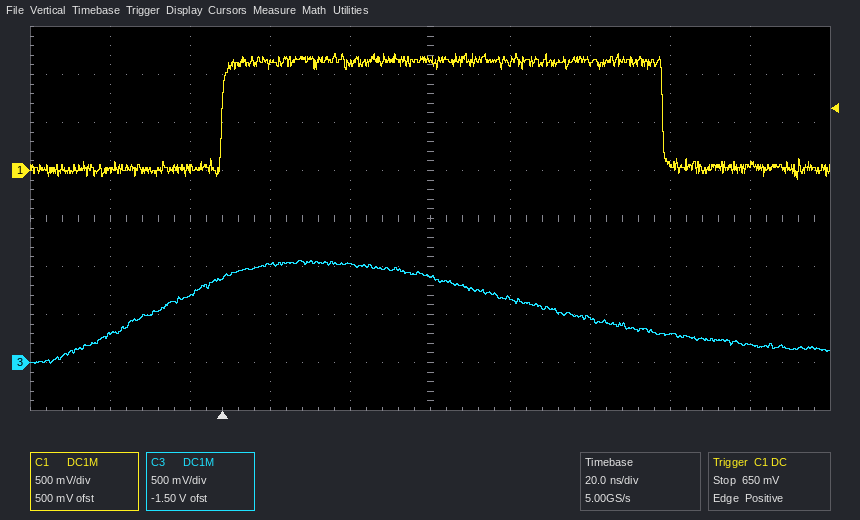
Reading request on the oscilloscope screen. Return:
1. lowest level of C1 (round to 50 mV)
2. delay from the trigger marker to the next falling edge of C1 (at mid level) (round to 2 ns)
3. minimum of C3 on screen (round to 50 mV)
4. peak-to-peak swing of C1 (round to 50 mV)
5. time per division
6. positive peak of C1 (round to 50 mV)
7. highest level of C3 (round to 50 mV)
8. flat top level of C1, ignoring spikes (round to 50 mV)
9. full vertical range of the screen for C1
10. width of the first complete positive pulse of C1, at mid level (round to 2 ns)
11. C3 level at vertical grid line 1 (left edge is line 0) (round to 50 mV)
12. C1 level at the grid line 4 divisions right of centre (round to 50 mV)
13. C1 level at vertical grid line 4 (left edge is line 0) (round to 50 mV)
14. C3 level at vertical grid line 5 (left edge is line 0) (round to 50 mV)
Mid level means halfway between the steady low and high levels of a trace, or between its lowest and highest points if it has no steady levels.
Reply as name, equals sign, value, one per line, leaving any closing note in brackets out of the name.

lowest level of C1 = -100 mV
delay from the trigger marker to the next falling edge of C1 (at mid level) = 110 ns
minimum of C3 on screen = 0 mV
peak-to-peak swing of C1 = 1.30 V
time per division = 20 ns
positive peak of C1 = 1.20 V
highest level of C3 = 1.05 V
flat top level of C1, ignoring spikes = 1.15 V
full vertical range of the screen for C1 = 4 V
width of the first complete positive pulse of C1, at mid level = 110 ns
C3 level at vertical grid line 1 (left edge is line 0) = 300 mV
C1 level at the grid line 4 divisions right of centre = 50 mV
C1 level at vertical grid line 4 (left edge is line 0) = 1.10 V
C3 level at vertical grid line 5 (left edge is line 0) = 900 mV
